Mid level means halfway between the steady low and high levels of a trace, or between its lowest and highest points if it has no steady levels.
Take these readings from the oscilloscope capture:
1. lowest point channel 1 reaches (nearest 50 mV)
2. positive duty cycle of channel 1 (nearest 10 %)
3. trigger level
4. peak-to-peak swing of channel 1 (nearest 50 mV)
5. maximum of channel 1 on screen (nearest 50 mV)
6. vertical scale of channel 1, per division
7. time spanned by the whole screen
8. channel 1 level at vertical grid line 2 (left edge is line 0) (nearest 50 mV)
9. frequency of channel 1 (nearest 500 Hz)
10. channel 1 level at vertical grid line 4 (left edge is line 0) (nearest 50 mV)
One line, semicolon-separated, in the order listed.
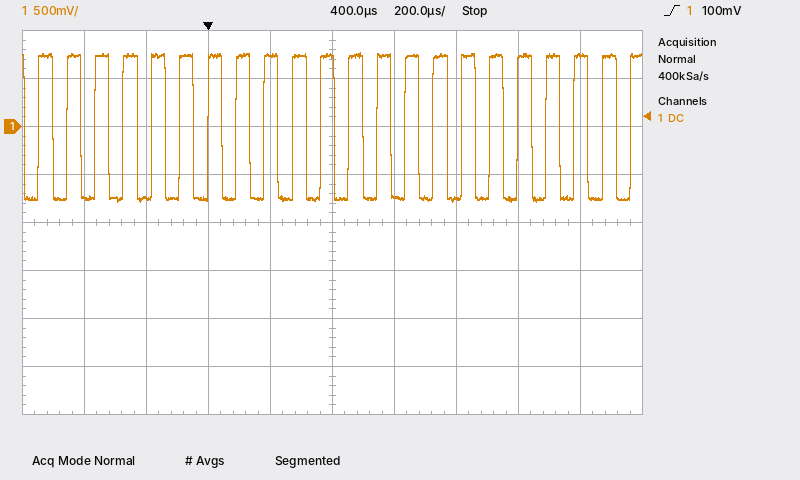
-800 mV; 50 %; 100 mV; 1.55 V; 750 mV; 500 mV; 2 ms; -750 mV; 11.0 kHz; 750 mV
